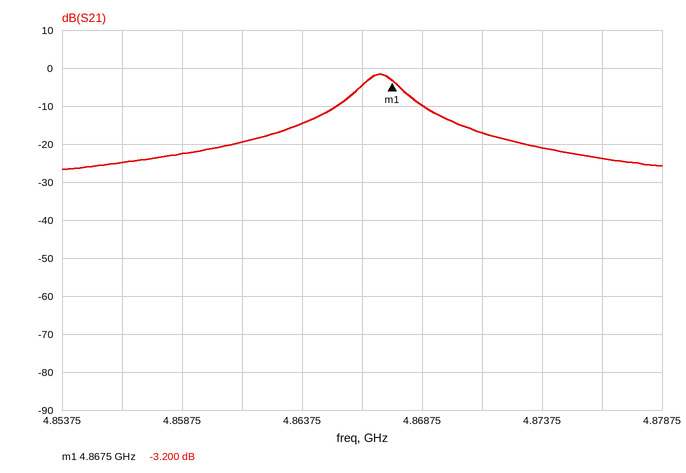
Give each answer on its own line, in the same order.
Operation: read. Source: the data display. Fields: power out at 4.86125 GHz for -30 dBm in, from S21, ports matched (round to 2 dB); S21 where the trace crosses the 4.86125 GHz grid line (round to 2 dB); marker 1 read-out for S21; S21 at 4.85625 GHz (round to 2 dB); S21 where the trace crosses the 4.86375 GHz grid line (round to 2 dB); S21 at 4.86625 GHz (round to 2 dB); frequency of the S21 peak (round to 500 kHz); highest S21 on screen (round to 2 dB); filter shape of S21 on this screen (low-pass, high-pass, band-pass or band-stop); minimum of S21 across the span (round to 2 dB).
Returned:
-50 dBm
-20 dB
-3.200 dB
-24 dB
-14 dB
-4 dB
4.8670 GHz
-2 dB
band-pass
-26 dB
